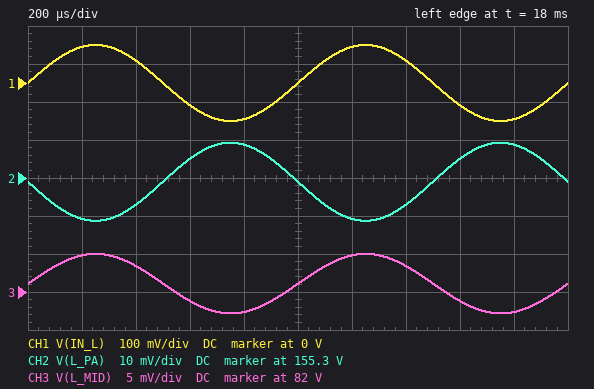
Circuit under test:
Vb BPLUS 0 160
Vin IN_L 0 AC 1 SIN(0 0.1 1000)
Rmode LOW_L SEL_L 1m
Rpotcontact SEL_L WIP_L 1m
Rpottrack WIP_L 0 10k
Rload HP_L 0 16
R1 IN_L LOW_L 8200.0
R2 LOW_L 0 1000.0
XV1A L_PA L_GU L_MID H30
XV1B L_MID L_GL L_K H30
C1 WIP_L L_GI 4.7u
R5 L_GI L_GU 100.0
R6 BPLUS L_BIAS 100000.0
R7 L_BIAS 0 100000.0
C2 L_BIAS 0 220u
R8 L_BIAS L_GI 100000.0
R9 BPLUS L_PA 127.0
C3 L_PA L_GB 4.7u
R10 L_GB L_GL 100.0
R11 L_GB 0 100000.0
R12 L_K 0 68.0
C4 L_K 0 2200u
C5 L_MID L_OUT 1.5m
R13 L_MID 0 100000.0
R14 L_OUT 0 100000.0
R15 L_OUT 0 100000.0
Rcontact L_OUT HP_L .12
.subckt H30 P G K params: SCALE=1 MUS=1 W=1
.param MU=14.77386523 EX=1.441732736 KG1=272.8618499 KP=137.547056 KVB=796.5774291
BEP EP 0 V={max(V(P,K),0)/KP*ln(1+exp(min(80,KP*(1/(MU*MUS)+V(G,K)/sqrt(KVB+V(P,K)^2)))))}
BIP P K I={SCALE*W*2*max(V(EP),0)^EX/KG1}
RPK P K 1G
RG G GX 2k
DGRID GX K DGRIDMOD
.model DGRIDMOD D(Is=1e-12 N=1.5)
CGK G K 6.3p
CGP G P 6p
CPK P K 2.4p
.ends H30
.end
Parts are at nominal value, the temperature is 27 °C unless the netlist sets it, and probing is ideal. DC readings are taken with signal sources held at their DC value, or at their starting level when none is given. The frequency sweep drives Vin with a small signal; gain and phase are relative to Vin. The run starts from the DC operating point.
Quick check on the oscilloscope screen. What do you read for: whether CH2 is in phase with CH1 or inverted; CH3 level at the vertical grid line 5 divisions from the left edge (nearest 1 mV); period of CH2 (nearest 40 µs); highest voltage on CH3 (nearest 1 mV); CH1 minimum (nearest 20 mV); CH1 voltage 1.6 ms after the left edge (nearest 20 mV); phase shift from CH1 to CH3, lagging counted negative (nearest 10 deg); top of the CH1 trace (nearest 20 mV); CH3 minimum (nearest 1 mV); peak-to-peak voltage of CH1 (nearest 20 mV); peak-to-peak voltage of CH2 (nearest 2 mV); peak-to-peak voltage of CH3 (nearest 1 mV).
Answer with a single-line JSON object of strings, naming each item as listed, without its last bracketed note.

{"whether CH2 is in phase with CH1 or inverted": "inverted", "CH3 level at the vertical grid line 5 divisions from the left edge": "82.001 V", "period of CH2": "1.00 ms", "highest voltage on CH3": "82.005 V", "CH1 minimum": "-100 mV", "CH1 voltage 1.6 ms after the left edge": "-60 mV", "phase shift from CH1 to CH3, lagging counted negative": "0 deg", "top of the CH1 trace": "100 mV", "CH3 minimum": "81.997 V", "peak-to-peak voltage of CH1": "200 mV", "peak-to-peak voltage of CH2": "20 mV", "peak-to-peak voltage of CH3": "8 mV"}
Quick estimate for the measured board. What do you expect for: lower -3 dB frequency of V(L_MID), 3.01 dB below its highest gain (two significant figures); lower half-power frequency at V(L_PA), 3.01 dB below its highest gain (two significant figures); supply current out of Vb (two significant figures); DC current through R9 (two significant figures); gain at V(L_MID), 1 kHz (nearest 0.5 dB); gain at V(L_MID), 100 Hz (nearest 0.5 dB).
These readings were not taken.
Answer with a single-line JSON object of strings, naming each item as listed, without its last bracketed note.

{"lower -3 dB frequency of V(L_MID), 3.01 dB below its highest gain": "260 mHz", "lower half-power frequency at V(L_PA), 3.01 dB below its highest gain": "2.6 Hz", "supply current out of Vb": "38 mA", "DC current through R9": "37 mA", "gain at V(L_MID), 1 kHz": "-28.0 dB", "gain at V(L_MID), 100 Hz": "-28.0 dB"}
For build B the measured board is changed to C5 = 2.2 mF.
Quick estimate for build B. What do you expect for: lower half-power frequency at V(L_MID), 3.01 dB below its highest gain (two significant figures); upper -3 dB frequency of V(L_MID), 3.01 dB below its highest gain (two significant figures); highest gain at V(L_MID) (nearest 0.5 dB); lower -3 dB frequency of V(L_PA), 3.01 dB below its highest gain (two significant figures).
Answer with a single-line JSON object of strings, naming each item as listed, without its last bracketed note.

{"lower half-power frequency at V(L_MID), 3.01 dB below its highest gain": "240 mHz", "upper -3 dB frequency of V(L_MID), 3.01 dB below its highest gain": "4.2 Hz", "highest gain at V(L_MID)": "-23.5 dB", "lower -3 dB frequency of V(L_PA), 3.01 dB below its highest gain": "1.6 Hz"}
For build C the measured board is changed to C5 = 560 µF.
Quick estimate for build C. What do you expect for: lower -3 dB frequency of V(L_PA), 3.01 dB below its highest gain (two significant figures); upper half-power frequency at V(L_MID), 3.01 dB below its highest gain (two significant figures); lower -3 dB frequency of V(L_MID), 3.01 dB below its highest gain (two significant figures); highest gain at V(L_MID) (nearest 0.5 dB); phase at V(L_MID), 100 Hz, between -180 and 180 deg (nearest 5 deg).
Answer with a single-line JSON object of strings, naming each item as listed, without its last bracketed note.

{"lower -3 dB frequency of V(L_PA), 3.01 dB below its highest gain": "7.8 Hz", "upper half-power frequency at V(L_MID), 3.01 dB below its highest gain": "11 Hz", "lower -3 dB frequency of V(L_MID), 3.01 dB below its highest gain": "300 mHz", "highest gain at V(L_MID)": "-21.5 dB", "phase at V(L_MID), 100 Hz, between -180 and 180 deg": "-5 deg"}
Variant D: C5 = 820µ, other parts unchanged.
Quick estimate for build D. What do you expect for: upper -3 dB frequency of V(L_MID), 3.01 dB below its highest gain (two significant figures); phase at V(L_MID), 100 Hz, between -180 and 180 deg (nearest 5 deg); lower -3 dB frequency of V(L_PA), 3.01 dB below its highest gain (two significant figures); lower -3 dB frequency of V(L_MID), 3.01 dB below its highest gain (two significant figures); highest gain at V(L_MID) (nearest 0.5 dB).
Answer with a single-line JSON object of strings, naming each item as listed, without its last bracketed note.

{"upper -3 dB frequency of V(L_MID), 3.01 dB below its highest gain": "8.3 Hz", "phase at V(L_MID), 100 Hz, between -180 and 180 deg": "-5 deg", "lower -3 dB frequency of V(L_PA), 3.01 dB below its highest gain": "5.3 Hz", "lower -3 dB frequency of V(L_MID), 3.01 dB below its highest gain": "280 mHz", "highest gain at V(L_MID)": "-22.0 dB"}
